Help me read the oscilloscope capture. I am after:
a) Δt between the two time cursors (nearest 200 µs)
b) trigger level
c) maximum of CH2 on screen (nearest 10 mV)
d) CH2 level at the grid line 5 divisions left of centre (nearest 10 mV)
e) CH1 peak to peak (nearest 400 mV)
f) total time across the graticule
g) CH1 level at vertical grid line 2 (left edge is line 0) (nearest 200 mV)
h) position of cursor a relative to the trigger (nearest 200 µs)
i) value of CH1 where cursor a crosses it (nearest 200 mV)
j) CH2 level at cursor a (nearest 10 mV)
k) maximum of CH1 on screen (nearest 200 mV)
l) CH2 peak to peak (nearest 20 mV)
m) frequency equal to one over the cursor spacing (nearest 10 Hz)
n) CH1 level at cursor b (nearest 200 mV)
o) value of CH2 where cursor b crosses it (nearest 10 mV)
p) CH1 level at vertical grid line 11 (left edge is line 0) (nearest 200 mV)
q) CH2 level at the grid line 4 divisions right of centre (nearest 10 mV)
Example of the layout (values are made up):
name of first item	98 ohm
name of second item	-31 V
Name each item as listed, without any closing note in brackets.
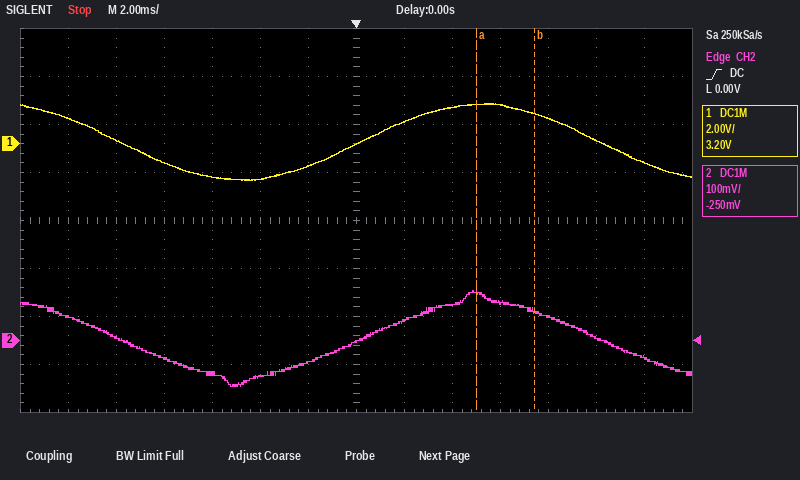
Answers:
Δt between the two time cursors	2.4 ms
trigger level	0.00 V
maximum of CH2 on screen	100 mV
CH2 level at the grid line 5 divisions left of centre	10 mV
CH1 peak to peak	3.2 V
total time across the graticule	28 ms
CH1 level at vertical grid line 2 (left edge is line 0)	200 mV
position of cursor a relative to the trigger	+5.0 ms
value of CH1 where cursor a crosses it	1.6 V
CH2 level at cursor a	100 mV
maximum of CH1 on screen	1.6 V
CH2 peak to peak	200 mV
frequency equal to one over the cursor spacing	420 Hz
CH1 level at cursor b	1.2 V
value of CH2 where cursor b crosses it	60 mV
CH1 level at vertical grid line 11 (left edge is line 0)	1.0 V
CH2 level at the grid line 4 divisions right of centre	50 mV
